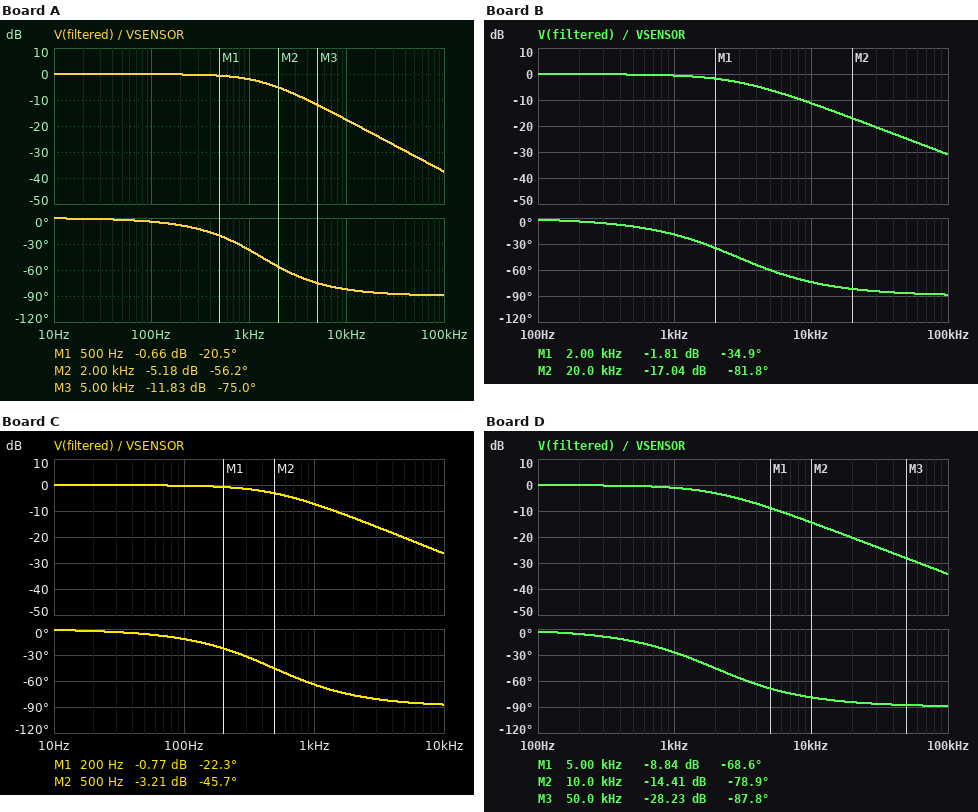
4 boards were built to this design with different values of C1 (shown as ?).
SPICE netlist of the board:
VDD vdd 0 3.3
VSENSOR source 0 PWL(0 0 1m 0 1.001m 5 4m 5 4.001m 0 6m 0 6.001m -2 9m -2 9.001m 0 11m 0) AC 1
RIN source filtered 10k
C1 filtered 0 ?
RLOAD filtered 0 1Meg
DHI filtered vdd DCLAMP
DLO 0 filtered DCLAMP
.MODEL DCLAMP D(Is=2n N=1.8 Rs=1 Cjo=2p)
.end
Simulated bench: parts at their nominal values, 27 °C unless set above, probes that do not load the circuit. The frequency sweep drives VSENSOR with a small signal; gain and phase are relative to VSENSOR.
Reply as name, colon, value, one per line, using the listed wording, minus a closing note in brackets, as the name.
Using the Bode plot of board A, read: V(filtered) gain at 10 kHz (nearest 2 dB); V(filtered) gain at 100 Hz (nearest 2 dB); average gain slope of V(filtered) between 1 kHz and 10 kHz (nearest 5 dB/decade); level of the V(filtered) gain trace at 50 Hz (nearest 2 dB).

V(filtered) gain at 10 kHz: -18 dB
V(filtered) gain at 100 Hz: 0 dB
average gain slope of V(filtered) between 1 kHz and 10 kHz: -15 dB/decade
level of the V(filtered) gain trace at 50 Hz: 0 dB
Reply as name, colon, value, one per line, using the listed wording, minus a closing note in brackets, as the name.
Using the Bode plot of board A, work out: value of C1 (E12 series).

value of C1: 12 nF
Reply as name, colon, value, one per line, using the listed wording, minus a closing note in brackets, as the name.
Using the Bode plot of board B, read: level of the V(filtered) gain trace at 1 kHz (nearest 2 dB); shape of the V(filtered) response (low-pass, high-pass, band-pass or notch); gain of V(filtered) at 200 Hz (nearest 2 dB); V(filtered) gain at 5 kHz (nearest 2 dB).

level of the V(filtered) gain trace at 1 kHz: 0 dB
shape of the V(filtered) response: low-pass
gain of V(filtered) at 200 Hz: 0 dB
V(filtered) gain at 5 kHz: -6 dB
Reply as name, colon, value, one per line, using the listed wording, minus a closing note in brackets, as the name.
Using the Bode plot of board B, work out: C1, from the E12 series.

C1, from the E12 series: 5.6 nF
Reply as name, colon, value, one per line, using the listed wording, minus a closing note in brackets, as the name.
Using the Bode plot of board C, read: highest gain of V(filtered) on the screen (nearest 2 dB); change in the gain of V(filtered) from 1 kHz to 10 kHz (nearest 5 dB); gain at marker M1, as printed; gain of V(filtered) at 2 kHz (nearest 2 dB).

highest gain of V(filtered) on the screen: 0 dB
change in the gain of V(filtered) from 1 kHz to 10 kHz: -20 dB
gain at marker M1, as printed: -0.77 dB
gain of V(filtered) at 2 kHz: -12 dB
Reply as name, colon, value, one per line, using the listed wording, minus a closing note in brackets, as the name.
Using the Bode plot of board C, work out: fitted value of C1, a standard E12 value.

fitted value of C1, a standard E12 value: 33 nF
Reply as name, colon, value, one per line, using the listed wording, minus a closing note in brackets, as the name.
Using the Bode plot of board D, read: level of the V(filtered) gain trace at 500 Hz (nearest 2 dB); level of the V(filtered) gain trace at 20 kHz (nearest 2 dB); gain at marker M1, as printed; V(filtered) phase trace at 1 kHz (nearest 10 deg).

level of the V(filtered) gain trace at 500 Hz: 0 dB
level of the V(filtered) gain trace at 20 kHz: -20 dB
gain at marker M1, as printed: -8.84 dB
V(filtered) phase trace at 1 kHz: -30 deg
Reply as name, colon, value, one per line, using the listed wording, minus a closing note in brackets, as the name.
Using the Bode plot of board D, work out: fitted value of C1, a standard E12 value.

fitted value of C1, a standard E12 value: 8.2 nF
